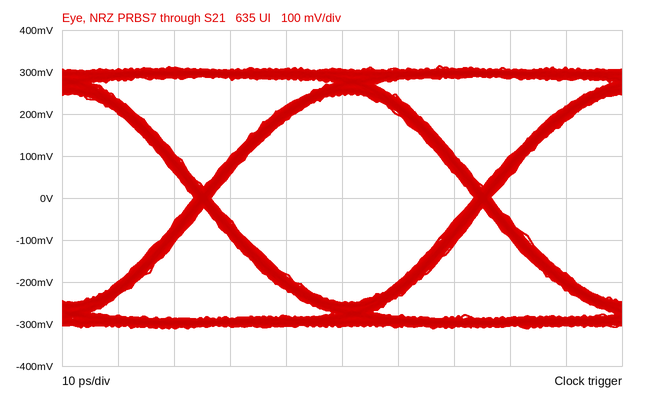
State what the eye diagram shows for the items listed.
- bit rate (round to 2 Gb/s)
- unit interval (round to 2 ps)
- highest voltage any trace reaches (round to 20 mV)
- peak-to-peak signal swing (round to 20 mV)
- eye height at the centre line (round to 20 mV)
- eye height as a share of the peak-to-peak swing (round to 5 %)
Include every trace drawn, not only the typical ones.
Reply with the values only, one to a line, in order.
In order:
20 Gb/s
50 ps
320 mV
620 mV
500 mV
80 %
